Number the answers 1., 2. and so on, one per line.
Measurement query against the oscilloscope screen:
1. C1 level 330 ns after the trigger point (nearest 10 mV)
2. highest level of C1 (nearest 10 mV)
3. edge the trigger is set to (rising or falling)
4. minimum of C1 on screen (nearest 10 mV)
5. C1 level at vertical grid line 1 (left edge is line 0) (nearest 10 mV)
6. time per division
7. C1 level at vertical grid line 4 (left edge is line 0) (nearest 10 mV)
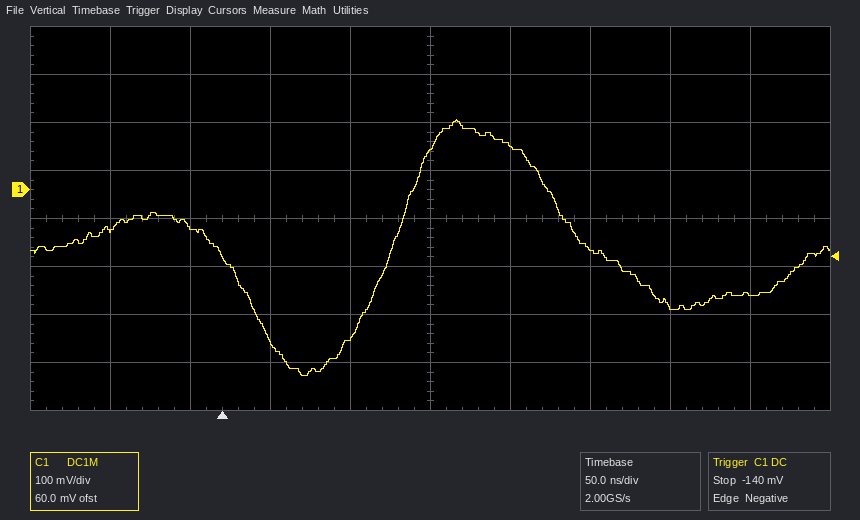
1. -220 mV
2. 150 mV
3. falling
4. -390 mV
5. -80 mV
6. 50 ns
7. -310 mV
